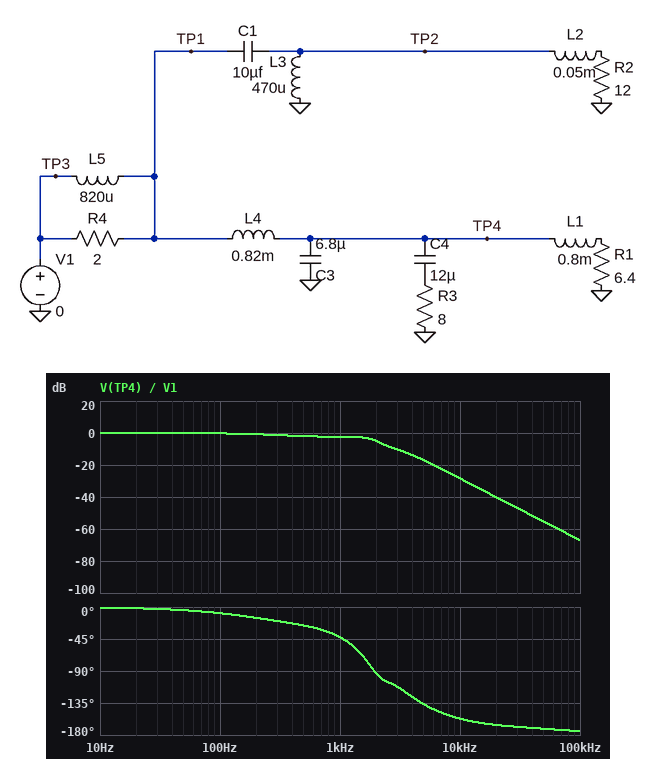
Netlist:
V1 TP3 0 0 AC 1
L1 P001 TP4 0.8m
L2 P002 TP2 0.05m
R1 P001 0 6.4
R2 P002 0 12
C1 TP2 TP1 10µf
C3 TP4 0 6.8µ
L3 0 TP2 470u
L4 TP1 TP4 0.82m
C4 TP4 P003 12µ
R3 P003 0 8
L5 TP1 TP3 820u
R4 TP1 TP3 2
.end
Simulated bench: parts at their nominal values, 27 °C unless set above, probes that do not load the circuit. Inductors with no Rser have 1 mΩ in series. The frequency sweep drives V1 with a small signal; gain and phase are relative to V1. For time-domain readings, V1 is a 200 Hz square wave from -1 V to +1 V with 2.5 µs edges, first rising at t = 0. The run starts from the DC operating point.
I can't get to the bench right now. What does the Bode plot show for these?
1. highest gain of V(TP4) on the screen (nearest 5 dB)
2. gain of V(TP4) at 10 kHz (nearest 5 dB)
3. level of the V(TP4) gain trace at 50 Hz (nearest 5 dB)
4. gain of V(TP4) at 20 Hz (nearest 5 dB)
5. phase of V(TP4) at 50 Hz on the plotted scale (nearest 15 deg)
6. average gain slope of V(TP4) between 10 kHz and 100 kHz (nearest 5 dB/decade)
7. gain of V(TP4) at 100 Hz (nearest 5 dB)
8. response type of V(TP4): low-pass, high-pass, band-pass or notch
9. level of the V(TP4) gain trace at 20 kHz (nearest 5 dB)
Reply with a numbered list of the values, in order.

1. 0 dB
2. -30 dB
3. 0 dB
4. 0 dB
5. 0 deg
6. -40 dB/decade
7. 0 dB
8. low-pass
9. -40 dB
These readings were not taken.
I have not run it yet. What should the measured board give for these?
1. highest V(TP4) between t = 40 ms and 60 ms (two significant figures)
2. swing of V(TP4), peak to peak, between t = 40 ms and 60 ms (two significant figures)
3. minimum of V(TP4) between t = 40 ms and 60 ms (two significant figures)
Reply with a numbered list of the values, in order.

1. 990 mV
2. 2.0 V
3. -990 mV
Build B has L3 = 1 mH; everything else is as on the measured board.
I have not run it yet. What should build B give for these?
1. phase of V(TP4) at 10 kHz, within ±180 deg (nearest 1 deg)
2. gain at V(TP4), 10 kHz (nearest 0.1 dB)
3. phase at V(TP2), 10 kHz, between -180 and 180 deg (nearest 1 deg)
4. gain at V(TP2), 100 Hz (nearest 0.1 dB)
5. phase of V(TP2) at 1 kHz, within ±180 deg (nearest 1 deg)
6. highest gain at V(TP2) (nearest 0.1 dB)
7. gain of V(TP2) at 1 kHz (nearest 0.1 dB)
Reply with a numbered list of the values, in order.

1. -159 deg
2. -28.3 dB
3. 12 deg
4. -48.3 dB
5. 133 deg
6. 0 dB
7. -7.9 dB
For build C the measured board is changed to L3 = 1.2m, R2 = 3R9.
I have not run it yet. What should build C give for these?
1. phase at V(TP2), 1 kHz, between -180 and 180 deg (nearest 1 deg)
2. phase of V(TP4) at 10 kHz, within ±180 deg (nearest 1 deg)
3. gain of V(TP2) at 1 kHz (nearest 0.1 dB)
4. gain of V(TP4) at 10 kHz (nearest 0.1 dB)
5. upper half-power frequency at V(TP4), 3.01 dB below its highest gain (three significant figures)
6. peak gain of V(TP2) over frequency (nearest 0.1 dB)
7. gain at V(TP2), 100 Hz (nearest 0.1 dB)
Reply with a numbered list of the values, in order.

1. 105 deg
2. -154 deg
3. -14.3 dB
4. -30.3 dB
5. 1.60 kHz
6. 0 dB
7. -46.8 dB
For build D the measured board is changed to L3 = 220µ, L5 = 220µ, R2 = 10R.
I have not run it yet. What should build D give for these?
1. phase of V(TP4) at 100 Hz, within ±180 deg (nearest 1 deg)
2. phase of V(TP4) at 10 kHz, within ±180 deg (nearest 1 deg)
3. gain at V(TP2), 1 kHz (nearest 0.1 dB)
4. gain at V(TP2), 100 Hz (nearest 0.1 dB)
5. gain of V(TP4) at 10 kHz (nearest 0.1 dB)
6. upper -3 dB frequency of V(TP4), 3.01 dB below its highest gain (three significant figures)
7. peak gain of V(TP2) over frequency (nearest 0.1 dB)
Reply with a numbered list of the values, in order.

1. -6 deg
2. -154 deg
3. -21.1 dB
4. -61.2 dB
5. -29.1 dB
6. 2.17 kHz
7. 1.6 dB
